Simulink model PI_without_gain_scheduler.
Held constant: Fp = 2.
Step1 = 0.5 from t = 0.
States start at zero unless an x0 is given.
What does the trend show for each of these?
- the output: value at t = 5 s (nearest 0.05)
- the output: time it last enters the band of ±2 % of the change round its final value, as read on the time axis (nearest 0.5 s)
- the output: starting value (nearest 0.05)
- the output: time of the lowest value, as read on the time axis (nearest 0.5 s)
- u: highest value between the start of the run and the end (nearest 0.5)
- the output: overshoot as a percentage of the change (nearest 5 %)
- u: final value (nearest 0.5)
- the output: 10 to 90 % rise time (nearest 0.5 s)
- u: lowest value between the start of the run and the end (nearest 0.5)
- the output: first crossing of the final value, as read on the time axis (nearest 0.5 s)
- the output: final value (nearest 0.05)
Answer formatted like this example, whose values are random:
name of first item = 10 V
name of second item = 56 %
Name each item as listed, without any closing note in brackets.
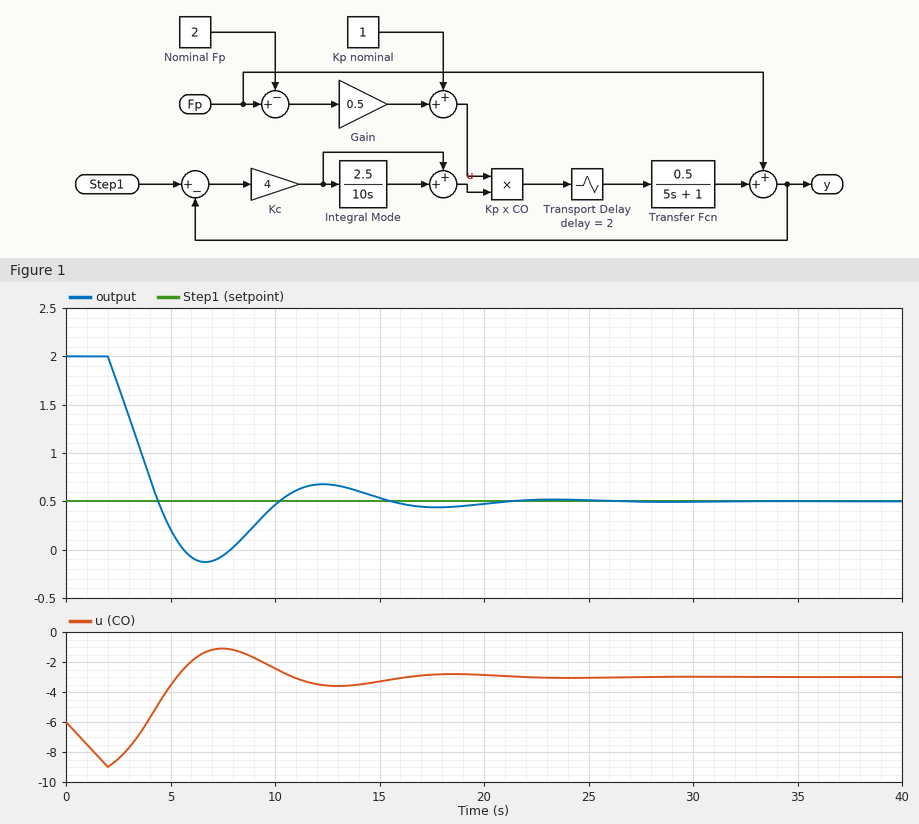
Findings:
the output: value at t = 5 s = 0.20
the output: time it last enters the band of ±2 % of the change round its final value, as read on the time axis = 20.0 s
the output: starting value = 2.00
the output: time of the lowest value, as read on the time axis = 6.5 s
u: highest value between the start of the run and the end = -1.0
the output: overshoot as a percentage of the change = 40 %
u: final value = -3.0
the output: 10 to 90 % rise time = 2.0 s
u: lowest value between the start of the run and the end = -9.0
the output: first crossing of the final value, as read on the time axis = 4.5 s
the output: final value = 0.50
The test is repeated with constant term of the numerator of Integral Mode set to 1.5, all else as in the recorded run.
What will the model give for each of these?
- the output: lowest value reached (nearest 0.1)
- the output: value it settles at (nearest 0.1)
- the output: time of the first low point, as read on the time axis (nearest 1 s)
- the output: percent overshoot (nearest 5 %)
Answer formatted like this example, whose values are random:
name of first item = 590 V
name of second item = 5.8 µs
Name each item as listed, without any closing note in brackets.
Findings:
the output: lowest value reached = 0.2
the output: value it settles at = 0.5
the output: time of the first low point, as read on the time axis = 6 s
the output: percent overshoot = 20 %
